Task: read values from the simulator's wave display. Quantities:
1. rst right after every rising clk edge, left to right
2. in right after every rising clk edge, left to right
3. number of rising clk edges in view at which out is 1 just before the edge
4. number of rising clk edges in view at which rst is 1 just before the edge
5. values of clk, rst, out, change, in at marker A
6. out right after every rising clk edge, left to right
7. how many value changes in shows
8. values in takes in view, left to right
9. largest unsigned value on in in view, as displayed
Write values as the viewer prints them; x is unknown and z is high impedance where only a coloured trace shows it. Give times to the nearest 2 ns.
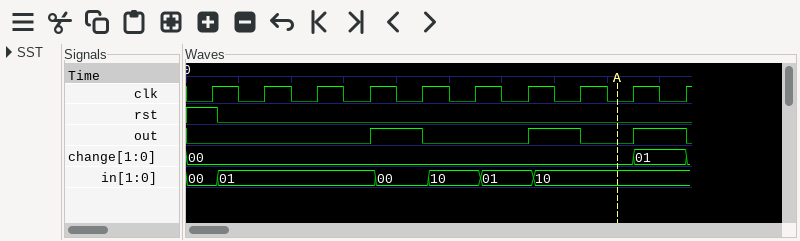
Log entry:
1 0 0 0 0 0 0 0 0 0
00, 01, 01, 01, 00, 10, 01, 10, 10, 10
3
1
clk=0, rst=0, out=0, change=00, in=10
0 0 0 1 0 0 1 0 1 0
5
00, 01, 00, 10, 01, 10
10
